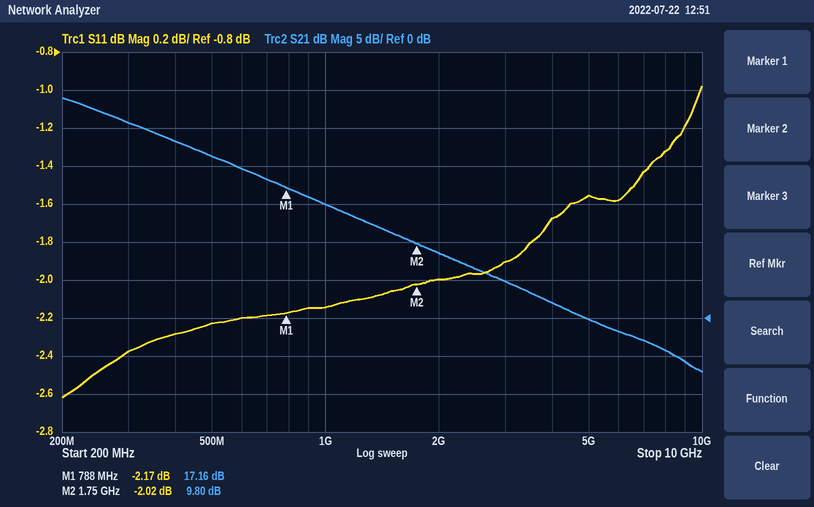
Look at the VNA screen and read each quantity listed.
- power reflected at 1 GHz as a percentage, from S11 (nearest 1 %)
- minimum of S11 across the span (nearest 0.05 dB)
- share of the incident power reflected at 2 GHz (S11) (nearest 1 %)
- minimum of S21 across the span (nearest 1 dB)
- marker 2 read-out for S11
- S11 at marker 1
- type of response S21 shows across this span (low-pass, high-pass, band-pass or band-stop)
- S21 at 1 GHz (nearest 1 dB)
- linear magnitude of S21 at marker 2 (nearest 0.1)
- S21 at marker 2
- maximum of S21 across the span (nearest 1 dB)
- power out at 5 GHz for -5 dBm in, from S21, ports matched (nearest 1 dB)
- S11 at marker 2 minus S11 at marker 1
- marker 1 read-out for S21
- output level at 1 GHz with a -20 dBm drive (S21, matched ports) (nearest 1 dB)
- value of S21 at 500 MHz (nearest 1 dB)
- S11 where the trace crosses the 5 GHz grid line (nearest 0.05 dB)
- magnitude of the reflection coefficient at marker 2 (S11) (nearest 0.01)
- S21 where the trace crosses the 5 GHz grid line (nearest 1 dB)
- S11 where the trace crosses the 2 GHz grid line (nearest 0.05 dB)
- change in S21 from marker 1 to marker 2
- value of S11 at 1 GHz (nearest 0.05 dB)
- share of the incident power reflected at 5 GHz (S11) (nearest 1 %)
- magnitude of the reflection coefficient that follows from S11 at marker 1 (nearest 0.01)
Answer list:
61 %
-2.60 dB
63 %
-7 dB
-2.02 dB
-2.17 dB
low-pass
15 dB
3.1
9.80 dB
29 dB
-5 dBm
0.15 dB
17.16 dB
-5 dBm
21 dB
-1.55 dB
0.79
0 dB
-2.00 dB
-7.36 dB
-2.15 dB
70 %
0.78
